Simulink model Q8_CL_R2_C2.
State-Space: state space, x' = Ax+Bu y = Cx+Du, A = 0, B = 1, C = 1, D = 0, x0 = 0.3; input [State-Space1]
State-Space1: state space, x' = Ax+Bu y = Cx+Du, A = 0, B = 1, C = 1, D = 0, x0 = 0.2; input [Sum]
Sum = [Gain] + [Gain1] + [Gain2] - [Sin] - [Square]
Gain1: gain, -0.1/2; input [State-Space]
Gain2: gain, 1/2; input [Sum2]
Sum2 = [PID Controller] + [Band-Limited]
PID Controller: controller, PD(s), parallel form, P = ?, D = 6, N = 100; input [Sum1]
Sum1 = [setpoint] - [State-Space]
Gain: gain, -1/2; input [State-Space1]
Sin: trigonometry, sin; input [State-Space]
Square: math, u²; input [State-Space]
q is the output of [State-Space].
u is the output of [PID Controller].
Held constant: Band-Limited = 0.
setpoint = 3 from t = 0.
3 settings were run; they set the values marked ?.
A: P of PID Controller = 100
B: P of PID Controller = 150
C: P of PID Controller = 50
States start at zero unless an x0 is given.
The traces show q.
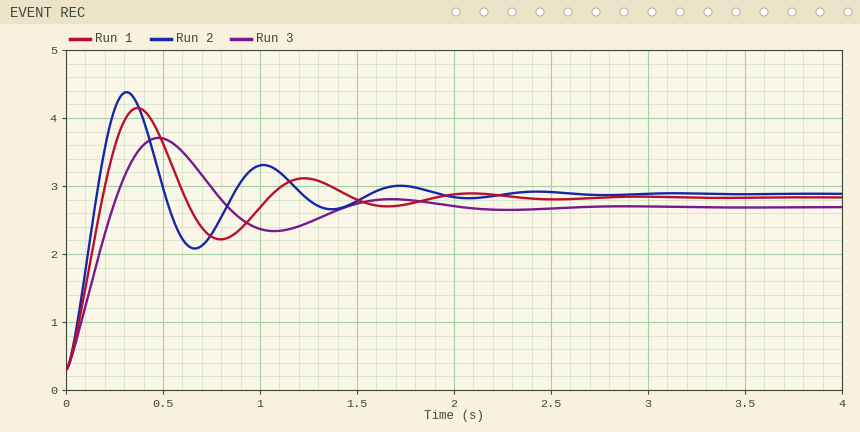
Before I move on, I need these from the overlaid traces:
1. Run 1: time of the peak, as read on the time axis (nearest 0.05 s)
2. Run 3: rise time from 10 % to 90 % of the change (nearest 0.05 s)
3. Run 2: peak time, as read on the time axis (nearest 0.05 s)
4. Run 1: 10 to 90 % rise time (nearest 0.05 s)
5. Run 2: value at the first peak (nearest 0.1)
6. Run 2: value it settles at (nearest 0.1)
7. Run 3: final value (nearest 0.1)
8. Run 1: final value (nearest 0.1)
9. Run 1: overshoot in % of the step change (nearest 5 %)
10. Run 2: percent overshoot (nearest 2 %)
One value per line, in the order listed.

0.35 s
0.20 s
0.30 s
0.15 s
4.4
2.9
2.7
2.8
50 %
58 %
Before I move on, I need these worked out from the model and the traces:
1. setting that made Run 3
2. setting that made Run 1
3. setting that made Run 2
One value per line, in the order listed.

C
A
B
